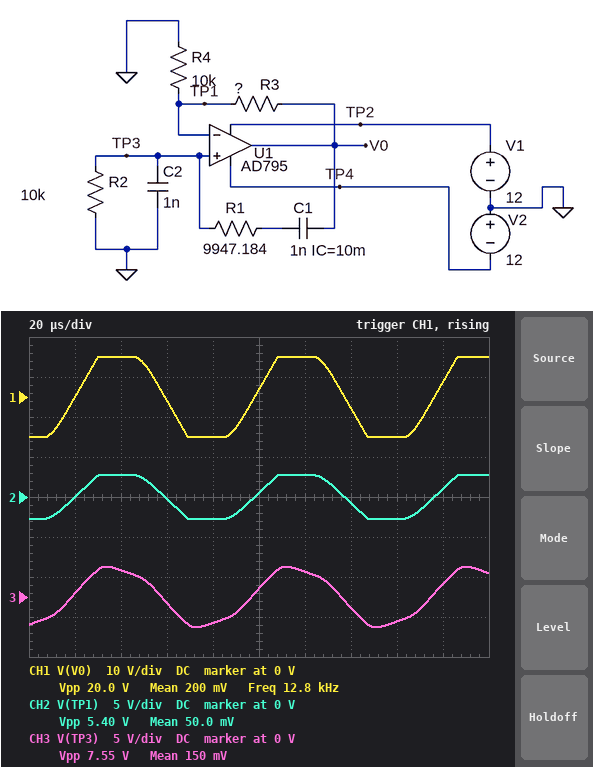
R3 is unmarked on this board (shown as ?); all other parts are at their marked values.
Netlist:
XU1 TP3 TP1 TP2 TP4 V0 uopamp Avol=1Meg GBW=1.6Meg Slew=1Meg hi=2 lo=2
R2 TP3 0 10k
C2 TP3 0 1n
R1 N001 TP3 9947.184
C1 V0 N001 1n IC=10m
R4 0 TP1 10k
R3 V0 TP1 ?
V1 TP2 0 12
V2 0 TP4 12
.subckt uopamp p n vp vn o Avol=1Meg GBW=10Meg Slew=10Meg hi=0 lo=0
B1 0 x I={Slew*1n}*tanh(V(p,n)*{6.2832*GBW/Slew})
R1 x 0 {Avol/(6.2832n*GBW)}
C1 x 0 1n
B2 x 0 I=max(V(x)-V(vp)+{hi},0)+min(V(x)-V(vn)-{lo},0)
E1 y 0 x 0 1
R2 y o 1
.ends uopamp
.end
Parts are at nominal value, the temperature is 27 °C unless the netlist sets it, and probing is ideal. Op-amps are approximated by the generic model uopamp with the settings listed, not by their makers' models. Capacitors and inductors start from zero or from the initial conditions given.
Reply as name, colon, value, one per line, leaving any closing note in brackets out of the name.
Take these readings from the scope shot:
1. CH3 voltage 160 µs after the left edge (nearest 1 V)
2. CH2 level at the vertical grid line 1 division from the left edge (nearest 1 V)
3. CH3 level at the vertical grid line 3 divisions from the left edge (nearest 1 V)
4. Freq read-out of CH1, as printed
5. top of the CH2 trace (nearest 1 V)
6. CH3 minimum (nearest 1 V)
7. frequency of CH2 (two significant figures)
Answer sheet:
CH3 voltage 160 µs after the left edge: -3 V
CH2 level at the vertical grid line 1 division from the left edge: 0 V
CH3 level at the vertical grid line 3 divisions from the left edge: -1 V
Freq read-out of CH1, as printed: 12.8 kHz
top of the CH2 trace: 3 V
CH3 minimum: -4 V
frequency of CH2: 13 kHz
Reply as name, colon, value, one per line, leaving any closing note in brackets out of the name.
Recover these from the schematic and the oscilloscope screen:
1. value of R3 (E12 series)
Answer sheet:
value of R3: 27 kΩ
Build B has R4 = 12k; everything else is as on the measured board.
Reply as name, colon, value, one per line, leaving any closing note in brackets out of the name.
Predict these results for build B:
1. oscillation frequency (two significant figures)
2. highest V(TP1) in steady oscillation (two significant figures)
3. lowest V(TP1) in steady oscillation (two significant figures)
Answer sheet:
oscillation frequency: 14 kHz
highest V(TP1) in steady oscillation: 3.1 V
lowest V(TP1) in steady oscillation: -3.1 V
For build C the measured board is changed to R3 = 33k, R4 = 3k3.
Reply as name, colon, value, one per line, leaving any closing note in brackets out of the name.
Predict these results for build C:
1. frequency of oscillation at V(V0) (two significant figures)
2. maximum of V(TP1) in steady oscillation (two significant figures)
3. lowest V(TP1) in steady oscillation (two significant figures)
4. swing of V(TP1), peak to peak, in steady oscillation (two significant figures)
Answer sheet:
frequency of oscillation at V(V0): 7.1 kHz
maximum of V(TP1) in steady oscillation: 910 mV
lowest V(TP1) in steady oscillation: -910 mV
swing of V(TP1), peak to peak, in steady oscillation: 1.8 V
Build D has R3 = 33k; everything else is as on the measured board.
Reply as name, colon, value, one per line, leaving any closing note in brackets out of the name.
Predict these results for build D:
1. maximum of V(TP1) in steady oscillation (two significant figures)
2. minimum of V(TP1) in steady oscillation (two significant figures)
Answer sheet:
maximum of V(TP1) in steady oscillation: 2.3 V
minimum of V(TP1) in steady oscillation: -2.3 V
